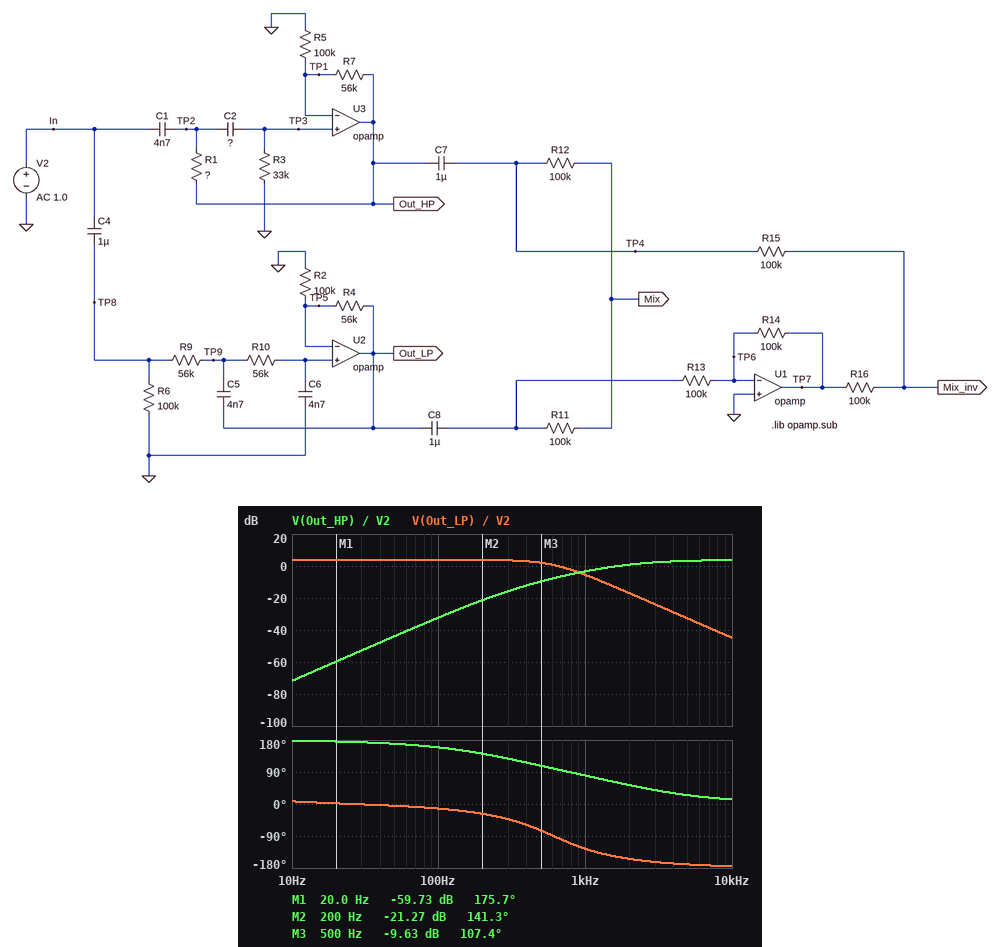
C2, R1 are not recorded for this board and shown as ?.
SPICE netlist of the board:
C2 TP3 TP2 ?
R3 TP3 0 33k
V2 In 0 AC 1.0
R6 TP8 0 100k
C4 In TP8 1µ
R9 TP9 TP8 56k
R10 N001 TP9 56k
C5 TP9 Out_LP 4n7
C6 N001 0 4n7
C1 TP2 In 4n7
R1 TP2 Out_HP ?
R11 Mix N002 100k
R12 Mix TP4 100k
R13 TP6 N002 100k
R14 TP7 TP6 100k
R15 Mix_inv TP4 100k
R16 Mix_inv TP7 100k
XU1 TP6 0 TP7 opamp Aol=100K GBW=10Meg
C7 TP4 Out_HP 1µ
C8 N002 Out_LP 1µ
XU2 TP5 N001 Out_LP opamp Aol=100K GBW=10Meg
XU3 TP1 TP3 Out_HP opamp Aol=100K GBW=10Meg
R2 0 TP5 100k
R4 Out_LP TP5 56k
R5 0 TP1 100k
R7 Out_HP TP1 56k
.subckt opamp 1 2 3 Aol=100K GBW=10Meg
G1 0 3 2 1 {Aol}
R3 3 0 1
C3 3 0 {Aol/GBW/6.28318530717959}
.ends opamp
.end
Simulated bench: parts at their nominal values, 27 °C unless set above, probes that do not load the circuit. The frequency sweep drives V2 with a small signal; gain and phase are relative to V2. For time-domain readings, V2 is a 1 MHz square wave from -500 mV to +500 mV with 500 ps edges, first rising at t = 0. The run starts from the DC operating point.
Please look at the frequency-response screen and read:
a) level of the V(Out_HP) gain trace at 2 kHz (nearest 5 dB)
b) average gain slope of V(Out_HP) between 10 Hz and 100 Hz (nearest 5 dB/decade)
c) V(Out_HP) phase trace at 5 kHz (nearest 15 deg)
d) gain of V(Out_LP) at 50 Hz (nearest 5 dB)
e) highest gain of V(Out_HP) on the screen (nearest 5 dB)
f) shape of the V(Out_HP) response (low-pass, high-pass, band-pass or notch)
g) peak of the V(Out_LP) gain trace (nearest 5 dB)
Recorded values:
0 dB
40 dB/decade
30 deg
5 dB
5 dB
high-pass
5 dB
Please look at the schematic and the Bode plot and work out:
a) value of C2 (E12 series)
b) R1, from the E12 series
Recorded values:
3.3 nF
82 kΩ
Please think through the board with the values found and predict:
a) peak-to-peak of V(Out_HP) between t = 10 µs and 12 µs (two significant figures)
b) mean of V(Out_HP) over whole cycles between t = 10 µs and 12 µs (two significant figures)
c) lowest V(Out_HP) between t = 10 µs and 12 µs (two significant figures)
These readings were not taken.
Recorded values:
1.6 V
670 mV
-120 mV
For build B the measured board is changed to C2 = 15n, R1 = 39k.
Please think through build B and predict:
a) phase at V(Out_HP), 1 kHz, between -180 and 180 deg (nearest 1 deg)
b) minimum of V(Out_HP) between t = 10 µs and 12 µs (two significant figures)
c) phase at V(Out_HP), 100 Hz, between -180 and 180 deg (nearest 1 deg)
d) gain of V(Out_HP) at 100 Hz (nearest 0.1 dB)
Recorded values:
50 deg
-50 mV
162 deg
-25.2 dB
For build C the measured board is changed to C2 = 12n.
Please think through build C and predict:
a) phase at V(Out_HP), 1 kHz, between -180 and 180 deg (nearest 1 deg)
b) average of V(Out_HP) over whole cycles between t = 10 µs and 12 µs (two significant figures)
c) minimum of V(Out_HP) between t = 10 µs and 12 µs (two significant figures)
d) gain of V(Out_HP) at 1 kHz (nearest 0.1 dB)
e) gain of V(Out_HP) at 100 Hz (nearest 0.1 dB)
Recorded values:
55 deg
720 mV
-68 mV
0.6 dB
-22.0 dB
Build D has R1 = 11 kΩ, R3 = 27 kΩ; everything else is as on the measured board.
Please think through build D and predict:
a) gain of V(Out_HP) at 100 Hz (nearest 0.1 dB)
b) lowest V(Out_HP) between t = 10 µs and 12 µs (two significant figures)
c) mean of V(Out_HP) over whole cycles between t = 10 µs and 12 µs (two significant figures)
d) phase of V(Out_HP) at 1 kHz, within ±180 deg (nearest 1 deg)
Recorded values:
-50.9 dB
-85 mV
700 mV
164 deg
